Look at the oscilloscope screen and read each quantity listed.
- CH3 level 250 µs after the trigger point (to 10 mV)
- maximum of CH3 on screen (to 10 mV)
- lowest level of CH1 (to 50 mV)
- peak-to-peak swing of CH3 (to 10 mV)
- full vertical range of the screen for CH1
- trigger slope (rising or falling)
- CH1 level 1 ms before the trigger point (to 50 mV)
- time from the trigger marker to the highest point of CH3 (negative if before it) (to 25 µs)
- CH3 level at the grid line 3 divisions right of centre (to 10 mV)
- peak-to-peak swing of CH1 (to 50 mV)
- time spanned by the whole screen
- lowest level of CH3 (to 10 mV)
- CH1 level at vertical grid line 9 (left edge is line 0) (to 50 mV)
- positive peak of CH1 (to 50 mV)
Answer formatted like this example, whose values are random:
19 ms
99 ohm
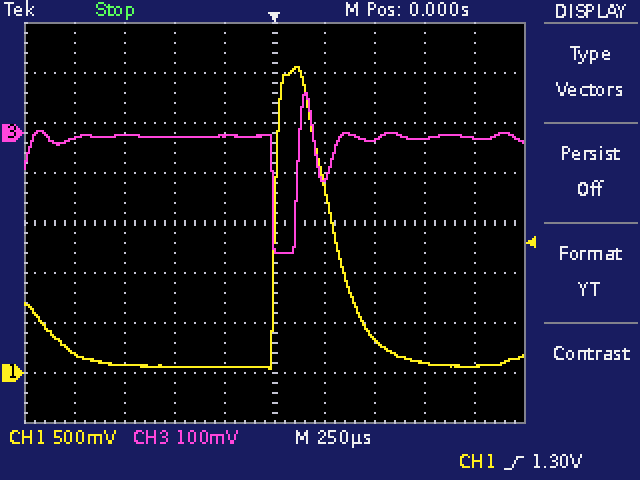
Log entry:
-90 mV
80 mV
50 mV
320 mV
4 V
rising
200 mV
+150 µs
-10 mV
3.00 V
2.5 ms
-240 mV
50 mV
3.05 V
